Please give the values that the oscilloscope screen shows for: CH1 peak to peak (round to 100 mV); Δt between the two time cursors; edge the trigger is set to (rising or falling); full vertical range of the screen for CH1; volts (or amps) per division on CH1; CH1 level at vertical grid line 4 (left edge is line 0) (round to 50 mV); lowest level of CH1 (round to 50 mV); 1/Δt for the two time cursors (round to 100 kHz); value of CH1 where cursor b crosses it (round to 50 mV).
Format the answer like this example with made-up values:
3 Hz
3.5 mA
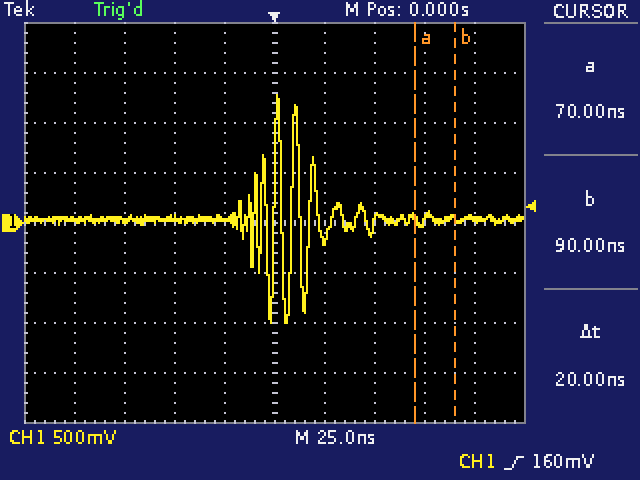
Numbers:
2.30 V
20 ns
rising
4 V
500 mV
50 mV
-1.00 V
50.0 MHz
50 mV
